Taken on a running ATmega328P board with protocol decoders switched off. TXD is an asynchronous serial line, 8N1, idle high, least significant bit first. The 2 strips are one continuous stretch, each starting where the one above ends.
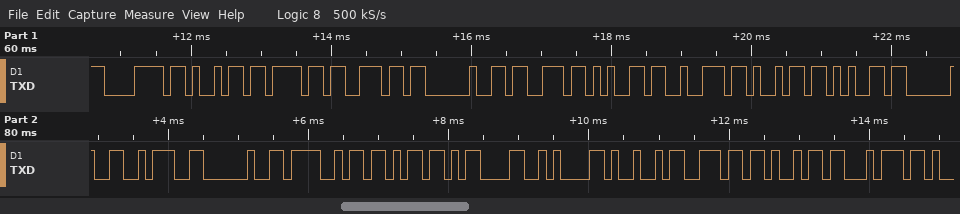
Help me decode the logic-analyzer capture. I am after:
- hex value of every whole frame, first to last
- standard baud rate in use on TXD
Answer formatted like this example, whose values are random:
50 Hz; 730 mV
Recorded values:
0x78 0x69 0x6F 0x6E 0x20 0x73 0x65 0x72 0x69 0x65 0x20 0x3A 0x20 0x4F 0x6B 0x0D 0x0A 0x49 0x6E 0x69 0x74; 9600 baud
